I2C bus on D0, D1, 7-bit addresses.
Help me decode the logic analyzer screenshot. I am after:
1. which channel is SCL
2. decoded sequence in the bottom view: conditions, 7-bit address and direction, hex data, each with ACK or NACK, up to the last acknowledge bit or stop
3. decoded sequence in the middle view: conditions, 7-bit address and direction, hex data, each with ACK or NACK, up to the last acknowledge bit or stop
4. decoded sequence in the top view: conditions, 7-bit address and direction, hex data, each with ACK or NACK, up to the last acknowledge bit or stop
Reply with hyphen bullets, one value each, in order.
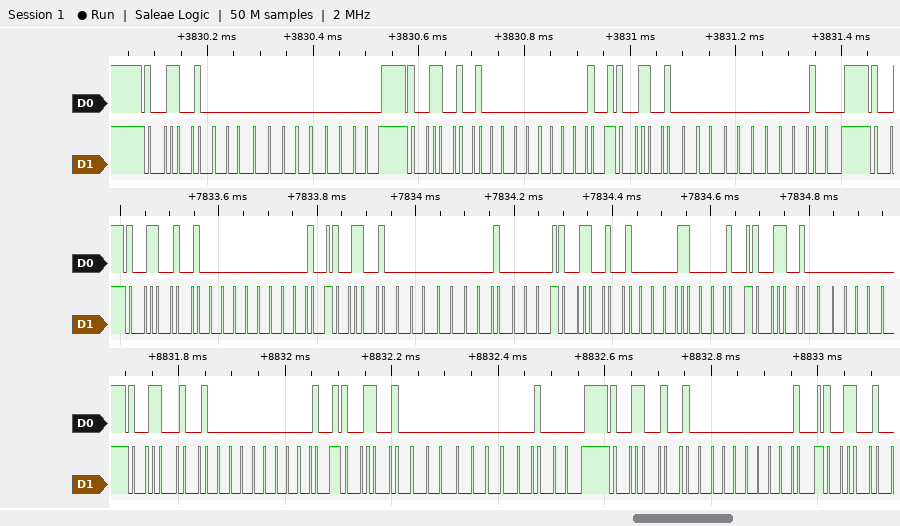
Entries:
- D1
- start, address 5A read ACK, 00 NACK, stop, start, address 5A write ACK, 02 ACK, stop, start, address 5A read ACK, 00 NACK, stop
- start, address 5A read ACK, 00 NACK, stop, start, address 5A write ACK, 04 ACK, stop, start, address 5A read ACK, 18 NACK, stop, start, address 5A write ACK
- start, address 5A write ACK, 00 ACK, stop, start, address 5A read ACK, 00 NACK, stop, start, address 5A write ACK, 01 ACK, stop
